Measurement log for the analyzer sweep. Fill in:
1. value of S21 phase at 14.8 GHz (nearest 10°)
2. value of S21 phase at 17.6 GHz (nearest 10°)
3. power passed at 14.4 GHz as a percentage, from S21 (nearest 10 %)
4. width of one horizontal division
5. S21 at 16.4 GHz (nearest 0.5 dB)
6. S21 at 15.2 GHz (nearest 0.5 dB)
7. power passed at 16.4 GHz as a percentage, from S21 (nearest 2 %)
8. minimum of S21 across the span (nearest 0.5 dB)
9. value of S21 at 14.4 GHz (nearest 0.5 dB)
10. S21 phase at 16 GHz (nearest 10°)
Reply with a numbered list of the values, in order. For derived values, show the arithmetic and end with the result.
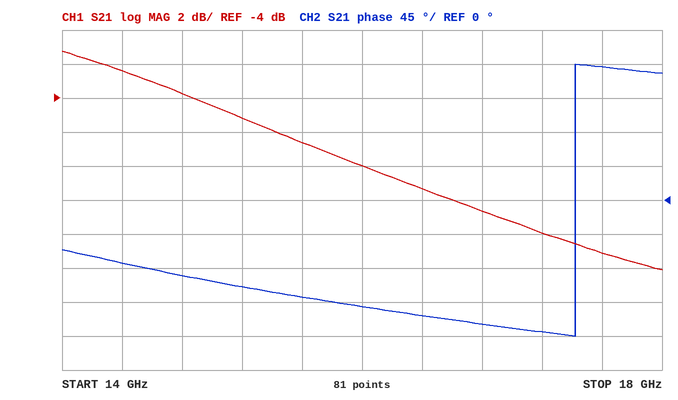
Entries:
1. -100°
2. 180°
3. 10^(-2.5/10) ≈ 56.2 %, so 60 % to the nearest 10 %
4. 400 MHz
5. -9.5 dB
6. -5.0 dB
7. 10^(-9.5/10) ≈ 11.2 %, so 12 % to the nearest 2 %
8. -14.0 dB
9. -2.5 dB
10. -140°
